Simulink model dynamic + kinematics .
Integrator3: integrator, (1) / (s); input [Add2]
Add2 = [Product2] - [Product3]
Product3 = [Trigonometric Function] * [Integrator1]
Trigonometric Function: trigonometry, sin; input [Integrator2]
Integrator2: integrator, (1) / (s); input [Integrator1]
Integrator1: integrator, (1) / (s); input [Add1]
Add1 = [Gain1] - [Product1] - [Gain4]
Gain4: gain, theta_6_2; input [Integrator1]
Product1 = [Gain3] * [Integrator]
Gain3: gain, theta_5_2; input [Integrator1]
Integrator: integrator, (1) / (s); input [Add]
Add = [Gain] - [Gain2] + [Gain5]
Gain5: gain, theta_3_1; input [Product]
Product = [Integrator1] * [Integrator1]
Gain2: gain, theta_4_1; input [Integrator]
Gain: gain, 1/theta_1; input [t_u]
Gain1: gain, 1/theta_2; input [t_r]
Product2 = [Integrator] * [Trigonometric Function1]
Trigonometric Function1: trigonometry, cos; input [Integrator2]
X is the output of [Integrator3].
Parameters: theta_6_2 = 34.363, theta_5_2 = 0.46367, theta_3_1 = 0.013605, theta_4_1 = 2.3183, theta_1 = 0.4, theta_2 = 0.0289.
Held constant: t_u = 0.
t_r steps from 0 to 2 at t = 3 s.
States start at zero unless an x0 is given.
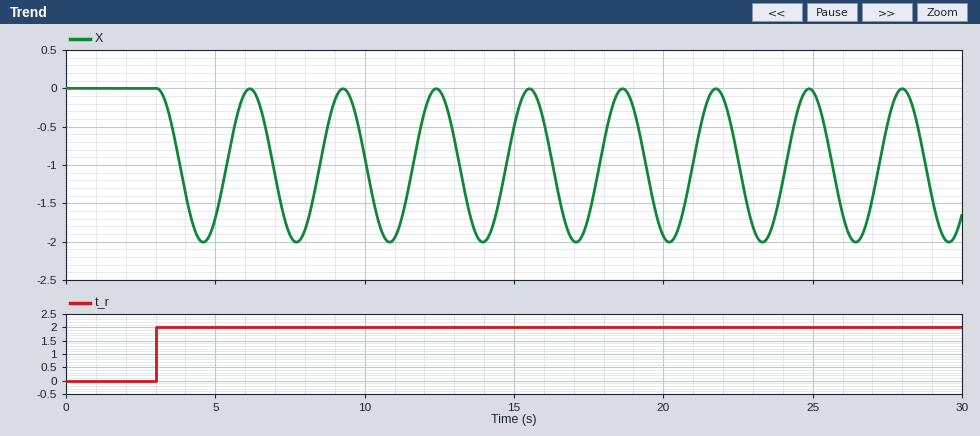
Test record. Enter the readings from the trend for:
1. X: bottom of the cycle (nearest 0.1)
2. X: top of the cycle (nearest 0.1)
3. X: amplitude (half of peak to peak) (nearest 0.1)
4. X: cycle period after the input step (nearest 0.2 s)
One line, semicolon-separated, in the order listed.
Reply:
-2.0; 0.0; 1.0; 3.2 s
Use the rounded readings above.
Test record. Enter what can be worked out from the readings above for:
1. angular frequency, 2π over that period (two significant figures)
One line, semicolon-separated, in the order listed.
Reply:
2.0 rad/s
